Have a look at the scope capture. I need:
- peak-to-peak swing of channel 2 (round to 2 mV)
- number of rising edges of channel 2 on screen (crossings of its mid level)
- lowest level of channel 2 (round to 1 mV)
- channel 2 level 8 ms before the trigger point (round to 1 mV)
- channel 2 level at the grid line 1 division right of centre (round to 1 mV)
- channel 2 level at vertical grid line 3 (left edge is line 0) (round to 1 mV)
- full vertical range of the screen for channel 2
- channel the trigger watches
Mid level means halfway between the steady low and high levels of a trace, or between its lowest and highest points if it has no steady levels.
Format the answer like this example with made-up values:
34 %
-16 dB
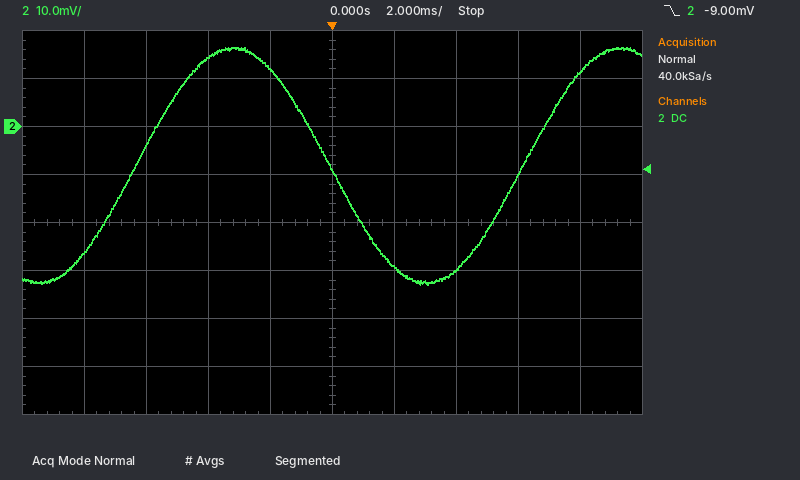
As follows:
50 mV
2
-33 mV
-26 mV
-29 mV
14 mV
80 mV
channel 2
